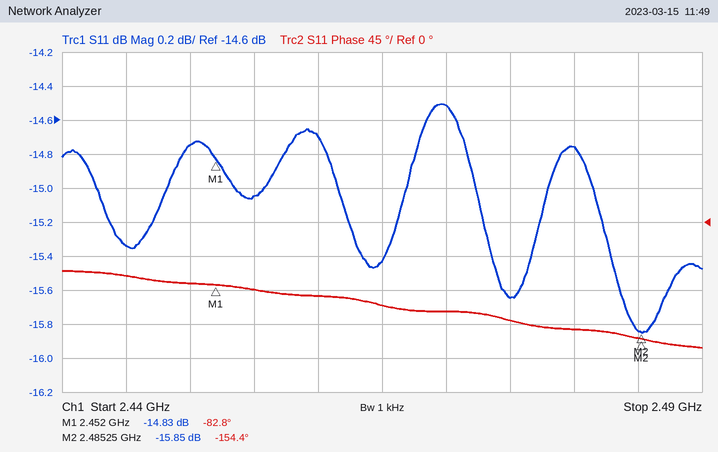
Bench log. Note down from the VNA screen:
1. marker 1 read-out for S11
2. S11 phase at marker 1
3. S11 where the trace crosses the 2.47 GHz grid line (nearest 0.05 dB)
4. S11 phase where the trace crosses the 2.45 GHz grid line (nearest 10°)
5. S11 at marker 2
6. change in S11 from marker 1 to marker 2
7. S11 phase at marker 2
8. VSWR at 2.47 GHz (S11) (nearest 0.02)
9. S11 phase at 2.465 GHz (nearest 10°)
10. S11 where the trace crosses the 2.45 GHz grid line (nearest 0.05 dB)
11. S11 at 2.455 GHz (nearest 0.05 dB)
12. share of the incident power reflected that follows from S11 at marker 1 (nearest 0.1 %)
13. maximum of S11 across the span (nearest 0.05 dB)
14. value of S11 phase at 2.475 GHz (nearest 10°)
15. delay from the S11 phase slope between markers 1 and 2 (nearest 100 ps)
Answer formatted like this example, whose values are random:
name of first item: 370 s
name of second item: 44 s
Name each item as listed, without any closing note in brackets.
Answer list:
marker 1 read-out for S11: -14.83 dB
S11 phase at marker 1: -82.8°
S11 where the trace crosses the 2.47 GHz grid line: -14.50 dB
S11 phase where the trace crosses the 2.45 GHz grid line: -80°
S11 at marker 2: -15.85 dB
change in S11 from marker 1 to marker 2: -1.02 dB
S11 phase at marker 2: -154.4°
VSWR at 2.47 GHz (S11): 1.46
S11 phase at 2.465 GHz: -110°
S11 where the trace crosses the 2.45 GHz grid line: -14.75 dB
S11 at 2.455 GHz: -15.05 dB
share of the incident power reflected that follows from S11 at marker 1: 3.3 %
maximum of S11 across the span: -14.50 dB
value of S11 phase at 2.475 GHz: -130°
delay from the S11 phase slope between markers 1 and 2: 6.0 ns
